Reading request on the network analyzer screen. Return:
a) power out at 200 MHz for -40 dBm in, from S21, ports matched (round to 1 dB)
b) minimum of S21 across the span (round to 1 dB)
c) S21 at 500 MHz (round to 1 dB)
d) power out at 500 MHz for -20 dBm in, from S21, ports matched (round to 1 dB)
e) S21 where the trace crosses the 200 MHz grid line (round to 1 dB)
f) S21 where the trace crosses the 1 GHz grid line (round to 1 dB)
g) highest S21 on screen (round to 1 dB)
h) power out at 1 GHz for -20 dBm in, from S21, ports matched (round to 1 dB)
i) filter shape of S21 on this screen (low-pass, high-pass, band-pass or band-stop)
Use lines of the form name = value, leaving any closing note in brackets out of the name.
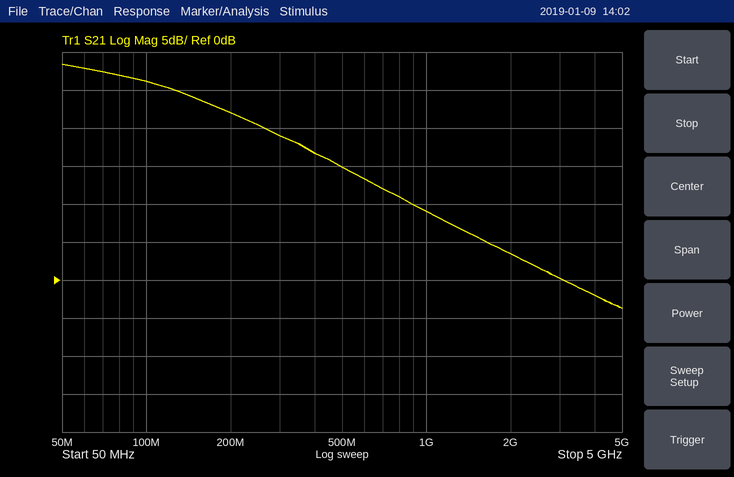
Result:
power out at 200 MHz for -40 dBm in, from S21, ports matched = -18 dBm
minimum of S21 across the span = -4 dB
S21 at 500 MHz = 15 dB
power out at 500 MHz for -20 dBm in, from S21, ports matched = -5 dBm
S21 where the trace crosses the 200 MHz grid line = 22 dB
S21 where the trace crosses the 1 GHz grid line = 9 dB
highest S21 on screen = 28 dB
power out at 1 GHz for -20 dBm in, from S21, ports matched = -11 dBm
filter shape of S21 on this screen = low-pass
